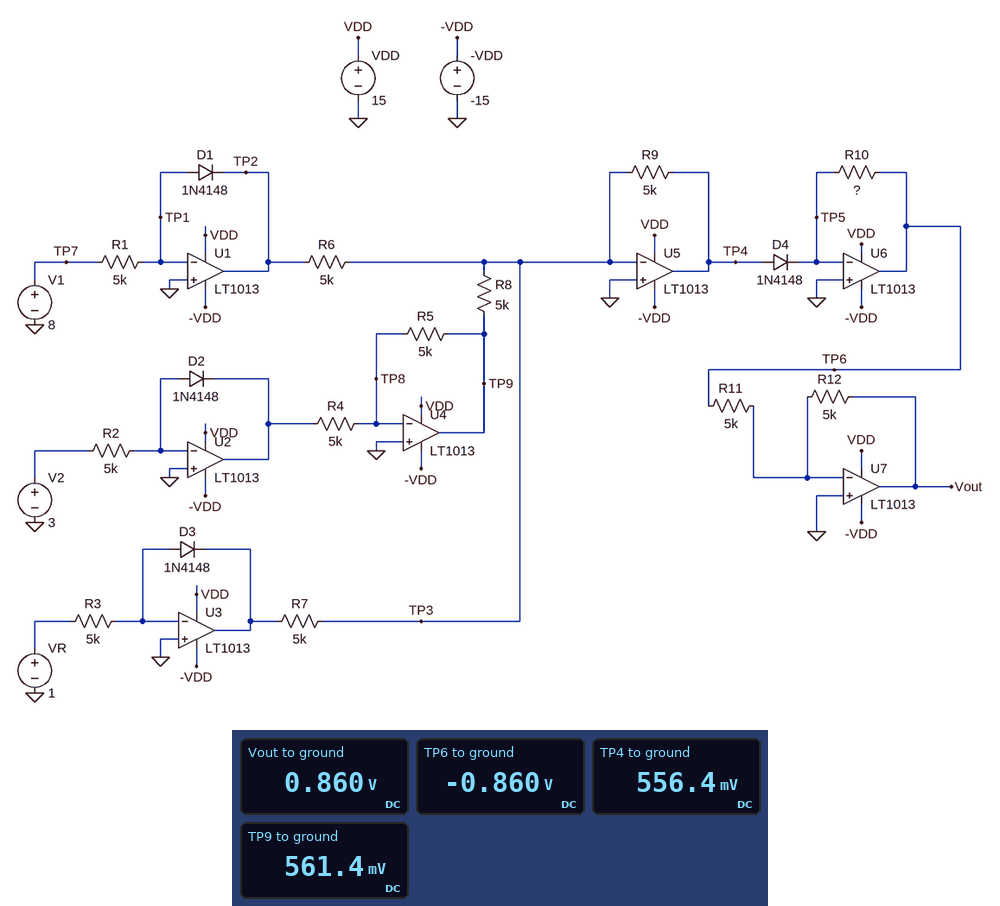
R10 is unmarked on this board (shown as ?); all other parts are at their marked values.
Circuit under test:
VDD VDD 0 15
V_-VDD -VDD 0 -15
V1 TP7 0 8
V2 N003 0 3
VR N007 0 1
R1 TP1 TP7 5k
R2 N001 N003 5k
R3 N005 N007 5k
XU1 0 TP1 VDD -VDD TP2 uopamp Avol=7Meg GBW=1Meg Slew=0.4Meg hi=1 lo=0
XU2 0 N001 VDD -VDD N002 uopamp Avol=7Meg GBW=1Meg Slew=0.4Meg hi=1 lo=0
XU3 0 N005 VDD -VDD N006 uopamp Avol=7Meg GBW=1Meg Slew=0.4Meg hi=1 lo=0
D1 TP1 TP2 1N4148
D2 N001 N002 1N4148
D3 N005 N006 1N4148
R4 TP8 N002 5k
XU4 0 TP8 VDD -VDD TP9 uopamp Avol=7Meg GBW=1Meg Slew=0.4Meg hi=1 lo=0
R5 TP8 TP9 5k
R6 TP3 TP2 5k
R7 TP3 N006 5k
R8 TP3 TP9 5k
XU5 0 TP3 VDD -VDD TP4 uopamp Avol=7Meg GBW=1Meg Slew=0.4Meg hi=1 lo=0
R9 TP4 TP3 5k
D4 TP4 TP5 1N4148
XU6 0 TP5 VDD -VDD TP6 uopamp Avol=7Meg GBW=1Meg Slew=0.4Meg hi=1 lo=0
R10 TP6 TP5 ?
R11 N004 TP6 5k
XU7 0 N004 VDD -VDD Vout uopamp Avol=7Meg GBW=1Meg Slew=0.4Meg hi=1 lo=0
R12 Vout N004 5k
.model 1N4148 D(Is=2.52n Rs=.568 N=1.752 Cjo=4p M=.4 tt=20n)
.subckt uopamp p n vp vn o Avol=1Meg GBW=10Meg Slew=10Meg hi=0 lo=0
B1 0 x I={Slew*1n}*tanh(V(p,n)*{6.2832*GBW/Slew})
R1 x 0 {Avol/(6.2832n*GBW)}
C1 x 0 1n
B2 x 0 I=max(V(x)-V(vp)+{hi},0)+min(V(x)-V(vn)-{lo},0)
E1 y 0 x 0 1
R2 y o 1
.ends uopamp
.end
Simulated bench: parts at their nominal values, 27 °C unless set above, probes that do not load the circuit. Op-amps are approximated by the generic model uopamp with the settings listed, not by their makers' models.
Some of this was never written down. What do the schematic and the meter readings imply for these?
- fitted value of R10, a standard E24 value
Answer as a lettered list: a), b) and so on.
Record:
a) 1.6 kΩ
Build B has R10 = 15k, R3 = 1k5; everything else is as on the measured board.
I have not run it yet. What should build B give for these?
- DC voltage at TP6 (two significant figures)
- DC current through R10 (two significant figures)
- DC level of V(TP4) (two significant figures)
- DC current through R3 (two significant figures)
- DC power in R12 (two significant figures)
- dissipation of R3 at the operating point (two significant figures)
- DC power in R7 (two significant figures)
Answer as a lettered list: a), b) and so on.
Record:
a) -15 V
b) 1.0 mA
c) 610 mV
d) 670 µA
e) 42 mW
f) 670 µW
g) 64 µW
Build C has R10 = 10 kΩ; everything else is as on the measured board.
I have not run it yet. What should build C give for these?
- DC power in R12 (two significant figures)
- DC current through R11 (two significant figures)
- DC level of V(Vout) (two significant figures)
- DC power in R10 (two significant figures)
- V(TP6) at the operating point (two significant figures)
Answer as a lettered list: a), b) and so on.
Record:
a) 5.8 mW
b) 1.1 mA
c) 5.4 V
d) 2.9 mW
e) -5.4 V
